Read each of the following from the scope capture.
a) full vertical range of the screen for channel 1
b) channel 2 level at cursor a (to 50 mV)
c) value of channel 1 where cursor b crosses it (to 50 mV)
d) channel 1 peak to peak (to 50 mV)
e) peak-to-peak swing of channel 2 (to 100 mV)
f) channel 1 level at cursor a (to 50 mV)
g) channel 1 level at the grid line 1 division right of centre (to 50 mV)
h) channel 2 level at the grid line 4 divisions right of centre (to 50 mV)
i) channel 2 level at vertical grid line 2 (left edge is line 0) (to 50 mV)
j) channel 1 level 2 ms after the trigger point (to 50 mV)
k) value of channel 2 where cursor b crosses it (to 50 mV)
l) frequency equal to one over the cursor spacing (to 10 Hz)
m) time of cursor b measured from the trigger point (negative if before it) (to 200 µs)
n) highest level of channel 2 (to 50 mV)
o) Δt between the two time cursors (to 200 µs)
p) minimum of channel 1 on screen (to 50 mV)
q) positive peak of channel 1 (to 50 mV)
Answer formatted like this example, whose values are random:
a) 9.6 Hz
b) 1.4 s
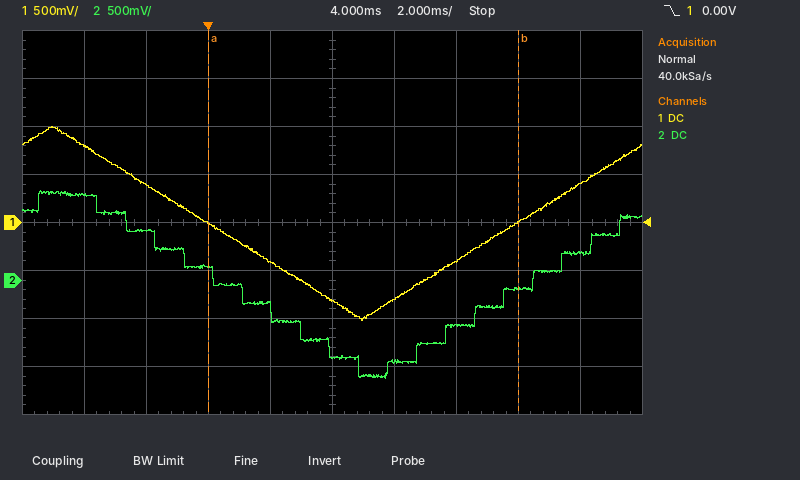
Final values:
a) 4 V
b) 150 mV
c) 0 mV
d) 2.00 V
e) 2.00 V
f) 0 mV
g) -800 mV
h) 300 mV
i) 500 mV
j) -400 mV
k) -100 mV
l) 100 Hz
m) +10.0 ms
n) 950 mV
o) 10.0 ms
p) -1.00 V
q) 1.00 V
